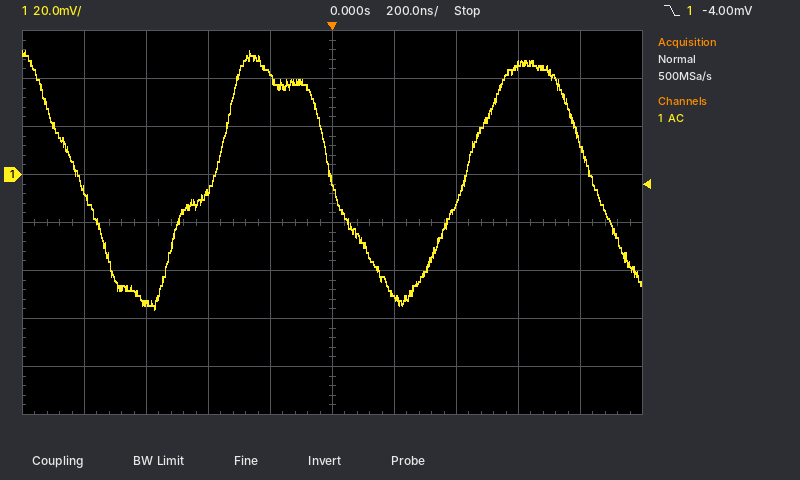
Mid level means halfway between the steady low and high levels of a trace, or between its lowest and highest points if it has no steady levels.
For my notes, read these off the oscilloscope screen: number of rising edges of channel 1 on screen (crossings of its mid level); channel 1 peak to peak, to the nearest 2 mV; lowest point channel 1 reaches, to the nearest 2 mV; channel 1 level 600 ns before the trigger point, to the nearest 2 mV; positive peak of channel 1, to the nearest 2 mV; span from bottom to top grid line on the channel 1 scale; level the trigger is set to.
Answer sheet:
2
108 mV
-56 mV
-54 mV
52 mV
160 mV
-4.00 mV
